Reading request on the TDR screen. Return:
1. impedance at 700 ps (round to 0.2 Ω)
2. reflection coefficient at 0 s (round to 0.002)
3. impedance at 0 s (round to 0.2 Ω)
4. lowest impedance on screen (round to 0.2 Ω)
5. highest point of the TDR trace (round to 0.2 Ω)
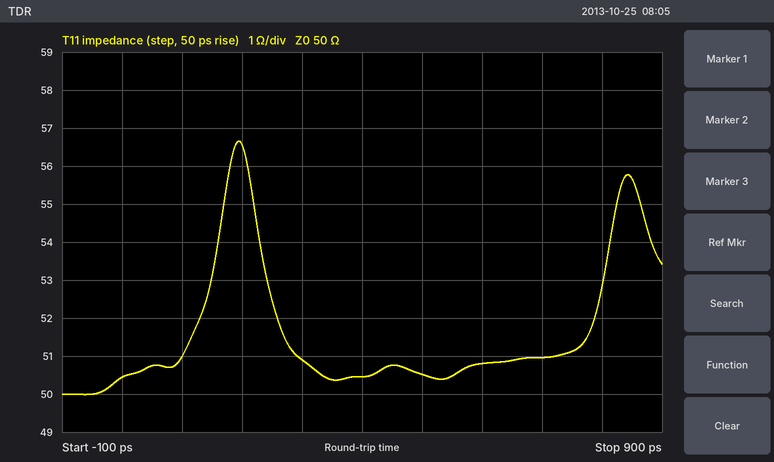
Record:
51.0 Ω
+0.004
50.4 Ω
50.0 Ω
56.6 Ω
